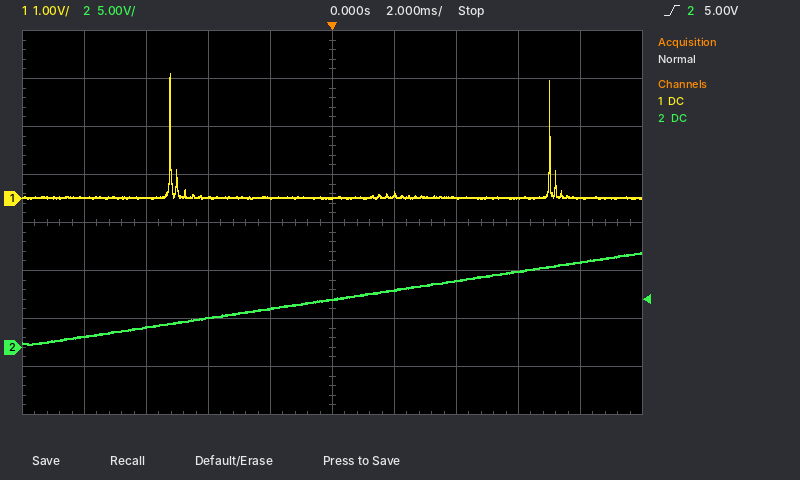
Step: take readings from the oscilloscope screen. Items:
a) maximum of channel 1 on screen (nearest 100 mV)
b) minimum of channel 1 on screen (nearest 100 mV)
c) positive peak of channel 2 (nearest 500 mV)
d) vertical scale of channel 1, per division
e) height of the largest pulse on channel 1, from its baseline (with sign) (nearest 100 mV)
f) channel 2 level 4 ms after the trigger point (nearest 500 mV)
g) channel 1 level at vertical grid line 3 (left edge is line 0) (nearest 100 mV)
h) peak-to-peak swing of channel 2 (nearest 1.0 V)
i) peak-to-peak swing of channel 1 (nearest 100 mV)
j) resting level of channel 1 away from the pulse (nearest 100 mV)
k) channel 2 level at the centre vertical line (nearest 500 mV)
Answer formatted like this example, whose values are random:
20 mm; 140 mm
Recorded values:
2.6 V; 0.0 V; 10.0 V; 1 V; +2.6 V; 7.0 V; 0.0 V; 10.0 V; 2.6 V; 0.0 V; 5.0 V
